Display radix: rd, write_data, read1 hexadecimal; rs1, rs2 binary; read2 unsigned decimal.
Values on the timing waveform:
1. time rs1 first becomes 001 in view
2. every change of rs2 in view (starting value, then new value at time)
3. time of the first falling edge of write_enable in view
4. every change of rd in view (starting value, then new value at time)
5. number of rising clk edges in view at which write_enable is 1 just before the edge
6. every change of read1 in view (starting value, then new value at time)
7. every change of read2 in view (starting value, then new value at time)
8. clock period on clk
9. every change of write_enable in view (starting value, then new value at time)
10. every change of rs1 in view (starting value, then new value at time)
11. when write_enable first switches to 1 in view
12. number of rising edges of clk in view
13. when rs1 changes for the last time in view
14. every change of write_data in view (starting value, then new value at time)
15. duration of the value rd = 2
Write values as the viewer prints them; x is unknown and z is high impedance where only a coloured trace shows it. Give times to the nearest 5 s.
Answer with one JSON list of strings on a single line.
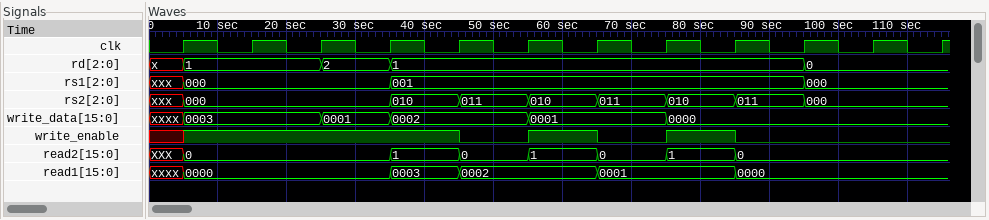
["35 s", "xxx, 000 at 5 s, 010 at 35 s, 011 at 45 s, 010 at 55 s, 011 at 65 s, 010 at 75 s, 011 at 85 s, 000 at 95 s", "45 s", "x, 1 at 5 s, 2 at 25 s, 1 at 35 s, 0 at 95 s", "6", "xxxx, 0000 at 5 s, 0003 at 35 s, 0002 at 45 s, 0001 at 65 s, 0000 at 85 s", "XXX, 0 at 5 s, 1 at 35 s, 0 at 45 s, 1 at 55 s, 0 at 65 s, 1 at 75 s, 0 at 85 s", "10 s", "x, 1 at 5 s, 0 at 45 s, 1 at 55 s, 0 at 65 s, 1 at 75 s, 0 at 85 s", "xxx, 000 at 5 s, 001 at 35 s, 000 at 95 s", "5 s", "12", "95 s", "xxxx, 0003 at 5 s, 0001 at 25 s, 0002 at 35 s, 0001 at 55 s, 0000 at 75 s", "10 s"]
